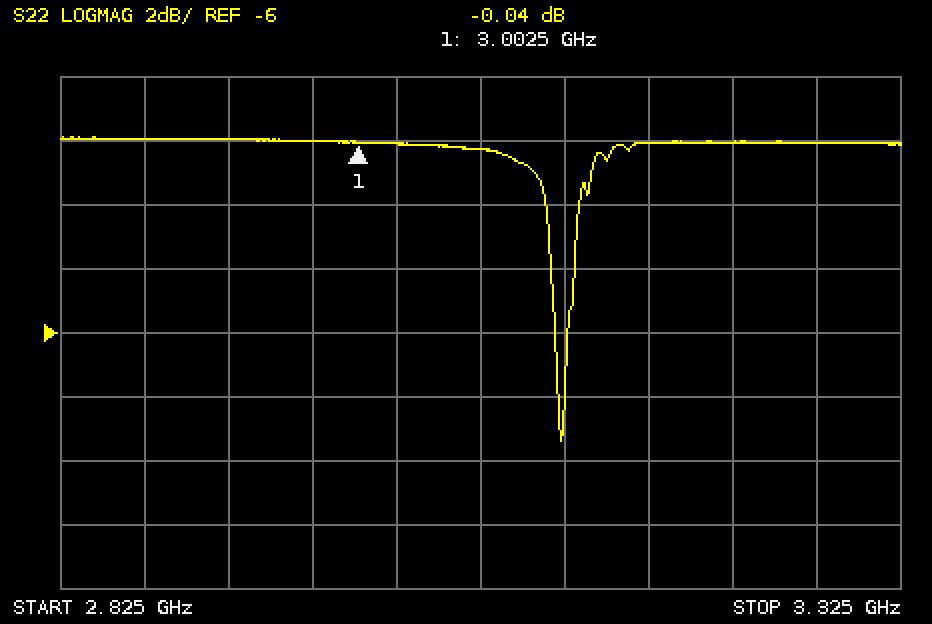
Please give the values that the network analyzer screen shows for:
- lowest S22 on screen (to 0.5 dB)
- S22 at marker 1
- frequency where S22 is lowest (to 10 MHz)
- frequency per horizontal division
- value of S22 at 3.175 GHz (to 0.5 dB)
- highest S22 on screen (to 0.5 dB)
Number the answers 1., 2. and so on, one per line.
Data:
1. -9.5 dB
2. -0.04 dB
3. 3.12 GHz
4. 50 MHz
5. 0.0 dB
6. 0.0 dB
